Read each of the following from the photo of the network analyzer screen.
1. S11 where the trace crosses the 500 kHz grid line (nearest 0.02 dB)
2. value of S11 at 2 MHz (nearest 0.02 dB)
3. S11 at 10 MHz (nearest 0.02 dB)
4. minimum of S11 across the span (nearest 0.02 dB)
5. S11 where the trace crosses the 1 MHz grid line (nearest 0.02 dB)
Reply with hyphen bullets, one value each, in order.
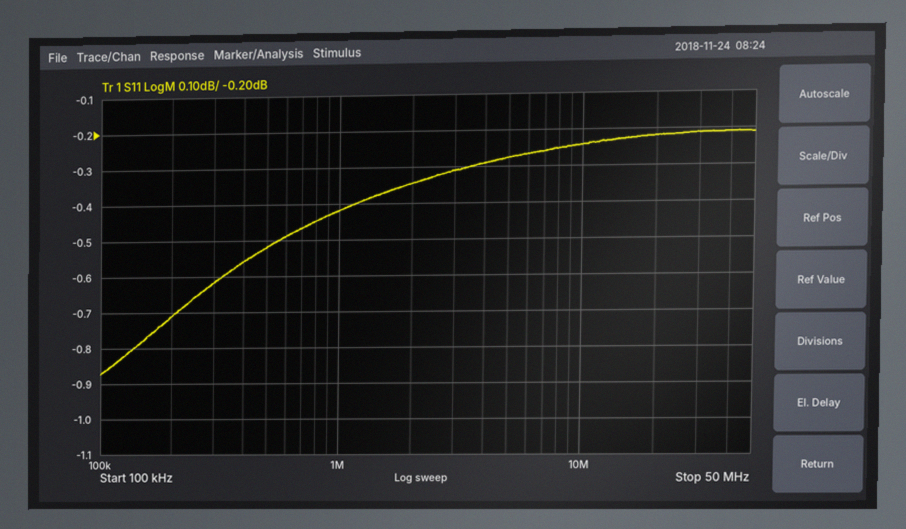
- -0.52 dB
- -0.34 dB
- -0.24 dB
- -0.88 dB
- -0.42 dB
